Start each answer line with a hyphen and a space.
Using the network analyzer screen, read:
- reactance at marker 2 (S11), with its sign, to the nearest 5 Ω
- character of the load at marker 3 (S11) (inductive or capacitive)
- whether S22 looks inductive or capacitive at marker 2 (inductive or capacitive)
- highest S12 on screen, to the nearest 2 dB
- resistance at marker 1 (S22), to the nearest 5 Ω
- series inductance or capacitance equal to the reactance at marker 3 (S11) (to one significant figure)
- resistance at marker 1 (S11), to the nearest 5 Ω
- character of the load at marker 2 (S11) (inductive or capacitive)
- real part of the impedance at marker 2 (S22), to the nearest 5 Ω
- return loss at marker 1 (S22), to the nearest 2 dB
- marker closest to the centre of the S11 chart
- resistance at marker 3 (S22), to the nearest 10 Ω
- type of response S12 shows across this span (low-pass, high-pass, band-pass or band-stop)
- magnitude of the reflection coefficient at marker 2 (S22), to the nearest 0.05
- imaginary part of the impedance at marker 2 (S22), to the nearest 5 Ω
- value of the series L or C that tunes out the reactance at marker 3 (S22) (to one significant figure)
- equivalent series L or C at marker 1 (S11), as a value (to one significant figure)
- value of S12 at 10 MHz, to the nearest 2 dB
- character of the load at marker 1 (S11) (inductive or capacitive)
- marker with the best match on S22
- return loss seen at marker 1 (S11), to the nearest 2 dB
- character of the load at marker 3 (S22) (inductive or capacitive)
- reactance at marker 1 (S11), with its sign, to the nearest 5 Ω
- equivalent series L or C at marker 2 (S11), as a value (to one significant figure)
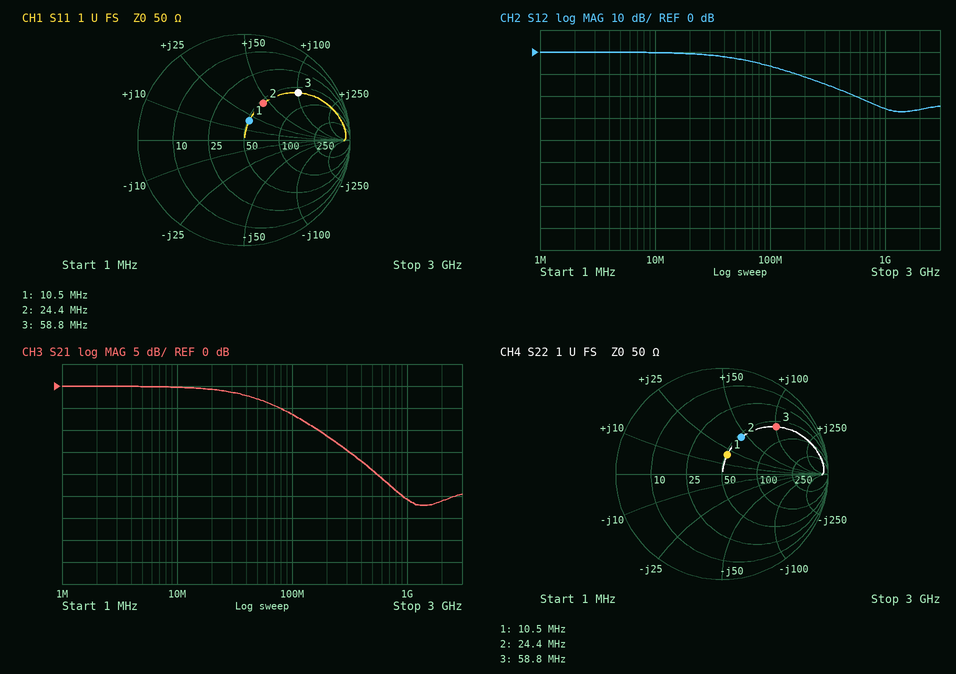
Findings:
- +45 Ω
- inductive
- inductive
- 0 dB
- 50 Ω
- 300 nH
- 50 Ω
- inductive
- 55 Ω
- 14 dB
- marker 1
- 60 Ω
- low-pass
- 0.40
- +45 Ω
- 30 pF
- 300 nH
- 0 dB
- inductive
- marker 1
- 14 dB
- inductive
- +20 Ω
- 300 nH
